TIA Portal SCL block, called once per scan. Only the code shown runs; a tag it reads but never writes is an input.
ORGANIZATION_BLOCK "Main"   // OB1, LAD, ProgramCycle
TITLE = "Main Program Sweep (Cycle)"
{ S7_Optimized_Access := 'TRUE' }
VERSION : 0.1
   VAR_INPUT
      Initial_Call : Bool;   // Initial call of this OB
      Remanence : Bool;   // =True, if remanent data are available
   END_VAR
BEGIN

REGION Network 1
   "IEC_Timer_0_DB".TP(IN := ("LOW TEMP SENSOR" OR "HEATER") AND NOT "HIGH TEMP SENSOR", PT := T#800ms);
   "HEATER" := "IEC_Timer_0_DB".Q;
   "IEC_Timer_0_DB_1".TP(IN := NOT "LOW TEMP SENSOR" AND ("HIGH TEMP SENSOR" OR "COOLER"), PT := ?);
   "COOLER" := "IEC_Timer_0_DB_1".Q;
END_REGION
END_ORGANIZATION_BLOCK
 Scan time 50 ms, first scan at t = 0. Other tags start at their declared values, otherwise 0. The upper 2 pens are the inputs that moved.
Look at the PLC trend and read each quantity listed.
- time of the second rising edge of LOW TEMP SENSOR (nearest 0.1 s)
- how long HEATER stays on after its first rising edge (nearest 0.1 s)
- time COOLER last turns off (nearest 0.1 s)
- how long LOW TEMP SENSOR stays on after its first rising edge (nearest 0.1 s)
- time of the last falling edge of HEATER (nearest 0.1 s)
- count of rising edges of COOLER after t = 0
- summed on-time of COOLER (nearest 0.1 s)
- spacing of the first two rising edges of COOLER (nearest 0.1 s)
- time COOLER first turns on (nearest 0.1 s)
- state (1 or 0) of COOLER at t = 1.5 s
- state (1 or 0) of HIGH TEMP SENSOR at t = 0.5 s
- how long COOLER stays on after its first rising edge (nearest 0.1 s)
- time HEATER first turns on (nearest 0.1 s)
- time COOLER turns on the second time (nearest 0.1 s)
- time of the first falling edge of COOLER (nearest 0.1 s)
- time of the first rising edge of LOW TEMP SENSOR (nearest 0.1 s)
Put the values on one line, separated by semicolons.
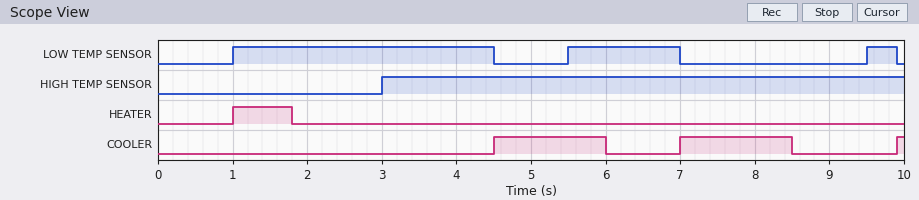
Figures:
5.5 s; 0.8 s; 8.5 s; 3.5 s; 1.8 s; 3; 3.1 s; 2.5 s; 4.5 s; 0; 0; 1.5 s; 1.0 s; 7.0 s; 6.0 s; 1.0 s
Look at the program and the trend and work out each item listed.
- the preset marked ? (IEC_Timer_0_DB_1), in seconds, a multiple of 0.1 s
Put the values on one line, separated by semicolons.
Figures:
1.5 s
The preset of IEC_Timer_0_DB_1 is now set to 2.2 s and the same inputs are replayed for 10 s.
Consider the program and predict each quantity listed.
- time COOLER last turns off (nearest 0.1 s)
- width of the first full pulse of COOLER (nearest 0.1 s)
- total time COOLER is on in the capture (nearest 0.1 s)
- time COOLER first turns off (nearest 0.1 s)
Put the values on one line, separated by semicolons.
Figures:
9.2 s; 2.2 s; 4.5 s; 6.7 s
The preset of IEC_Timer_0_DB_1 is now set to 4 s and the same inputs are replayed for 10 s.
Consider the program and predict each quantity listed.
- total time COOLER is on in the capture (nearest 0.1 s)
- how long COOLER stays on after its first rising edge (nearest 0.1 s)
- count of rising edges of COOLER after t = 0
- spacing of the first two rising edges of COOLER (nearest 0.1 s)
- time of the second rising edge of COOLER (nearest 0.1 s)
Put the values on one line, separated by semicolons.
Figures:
4.1 s; 4.0 s; 2; 5.4 s; 9.9 s
